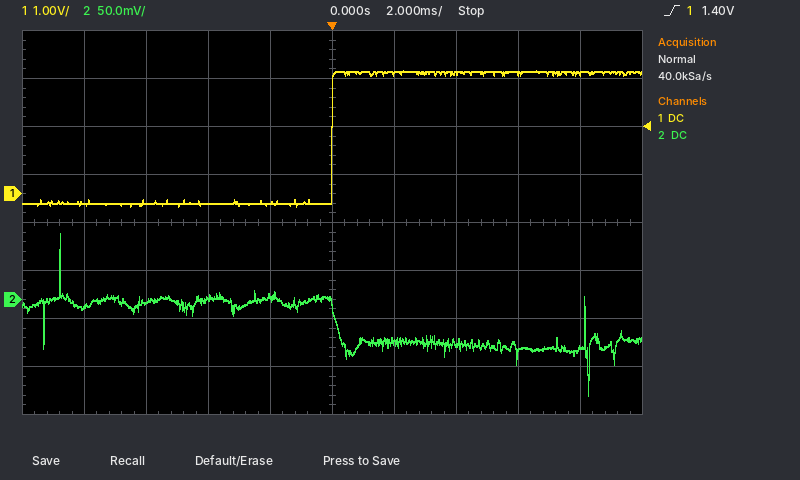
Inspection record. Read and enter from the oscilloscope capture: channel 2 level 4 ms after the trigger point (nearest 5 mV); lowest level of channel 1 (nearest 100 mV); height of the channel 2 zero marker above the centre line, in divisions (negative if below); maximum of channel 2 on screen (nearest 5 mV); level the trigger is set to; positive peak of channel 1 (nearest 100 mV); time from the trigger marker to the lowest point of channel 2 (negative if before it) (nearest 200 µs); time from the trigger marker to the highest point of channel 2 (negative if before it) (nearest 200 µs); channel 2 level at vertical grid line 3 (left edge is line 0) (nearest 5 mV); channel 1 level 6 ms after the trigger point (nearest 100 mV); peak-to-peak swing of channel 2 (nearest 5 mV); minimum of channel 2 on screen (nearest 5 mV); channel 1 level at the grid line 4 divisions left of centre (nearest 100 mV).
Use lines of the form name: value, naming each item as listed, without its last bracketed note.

channel 2 level 4 ms after the trigger point: -45 mV
lowest level of channel 1: -300 mV
height of the channel 2 zero marker above the centre line, in divisions: -1.6 div
maximum of channel 2 on screen: 70 mV
level the trigger is set to: 1.40 V
positive peak of channel 1: 2.6 V
time from the trigger marker to the lowest point of channel 2 (negative if before it): +8.2 ms
time from the trigger marker to the highest point of channel 2 (negative if before it): -8.8 ms
channel 2 level at vertical grid line 3 (left edge is line 0): 0 mV
channel 1 level 6 ms after the trigger point: 2.5 V
peak-to-peak swing of channel 2: 170 mV
minimum of channel 2 on screen: -100 mV
channel 1 level at the grid line 4 divisions left of centre: -200 mV
